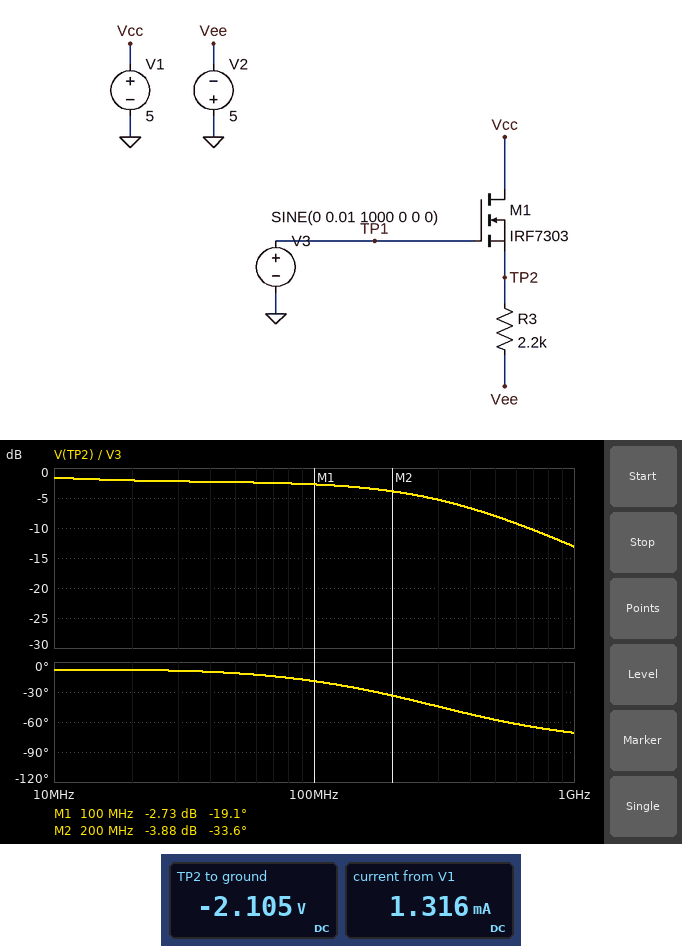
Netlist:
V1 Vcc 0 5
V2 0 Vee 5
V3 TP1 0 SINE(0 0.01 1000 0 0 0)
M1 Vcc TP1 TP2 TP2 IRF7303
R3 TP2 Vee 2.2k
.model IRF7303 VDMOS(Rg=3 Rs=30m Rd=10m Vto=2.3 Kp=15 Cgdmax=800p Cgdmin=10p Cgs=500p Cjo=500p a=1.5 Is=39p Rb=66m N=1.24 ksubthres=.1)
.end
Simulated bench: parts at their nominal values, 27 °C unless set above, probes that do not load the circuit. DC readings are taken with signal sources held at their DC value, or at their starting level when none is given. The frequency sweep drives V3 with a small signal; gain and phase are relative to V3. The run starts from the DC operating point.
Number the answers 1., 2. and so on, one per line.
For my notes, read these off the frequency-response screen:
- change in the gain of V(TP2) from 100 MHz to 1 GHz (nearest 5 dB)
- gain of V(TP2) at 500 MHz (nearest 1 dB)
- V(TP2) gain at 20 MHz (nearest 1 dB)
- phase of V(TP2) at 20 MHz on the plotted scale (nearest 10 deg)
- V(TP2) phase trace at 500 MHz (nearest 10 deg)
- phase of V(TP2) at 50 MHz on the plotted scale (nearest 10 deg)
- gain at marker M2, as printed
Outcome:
1. -10 dB
2. -8 dB
3. -2 dB
4. -10 deg
5. -60 deg
6. -10 deg
7. -3.88 dB
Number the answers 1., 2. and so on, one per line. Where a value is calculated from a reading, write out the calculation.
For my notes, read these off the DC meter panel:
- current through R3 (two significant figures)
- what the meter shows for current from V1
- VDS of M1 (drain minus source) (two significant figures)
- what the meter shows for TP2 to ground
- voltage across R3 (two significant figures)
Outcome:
1. (-2.105 V - (-5 V)) / 2.2 kΩ = 1.3 mA
2. 1.316 mA
3. 5 V - (-2.105 V) = 7.1 V
4. -2.105 V
5. -2.105 V - (-5 V) = 2.9 V
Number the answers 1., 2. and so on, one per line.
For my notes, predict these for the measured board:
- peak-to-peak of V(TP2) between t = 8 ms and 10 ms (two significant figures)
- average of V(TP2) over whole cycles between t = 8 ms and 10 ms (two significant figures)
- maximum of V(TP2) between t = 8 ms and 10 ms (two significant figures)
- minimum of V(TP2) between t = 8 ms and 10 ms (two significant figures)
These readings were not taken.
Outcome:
1. 20 mV
2. -2.1 V
3. -2.1 V
4. -2.1 V
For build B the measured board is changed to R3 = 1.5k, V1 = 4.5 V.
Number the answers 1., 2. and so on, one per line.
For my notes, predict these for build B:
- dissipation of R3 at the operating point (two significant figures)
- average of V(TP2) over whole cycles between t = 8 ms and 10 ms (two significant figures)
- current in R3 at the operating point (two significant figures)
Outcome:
1. 5.5 mW
2. -2.1 V
3. 1.9 mA
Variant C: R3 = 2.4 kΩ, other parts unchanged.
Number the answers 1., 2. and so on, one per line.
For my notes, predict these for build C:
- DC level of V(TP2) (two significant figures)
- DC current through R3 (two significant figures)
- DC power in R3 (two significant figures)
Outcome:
1. -2.1 V
2. 1.2 mA
3. 3.5 mW
